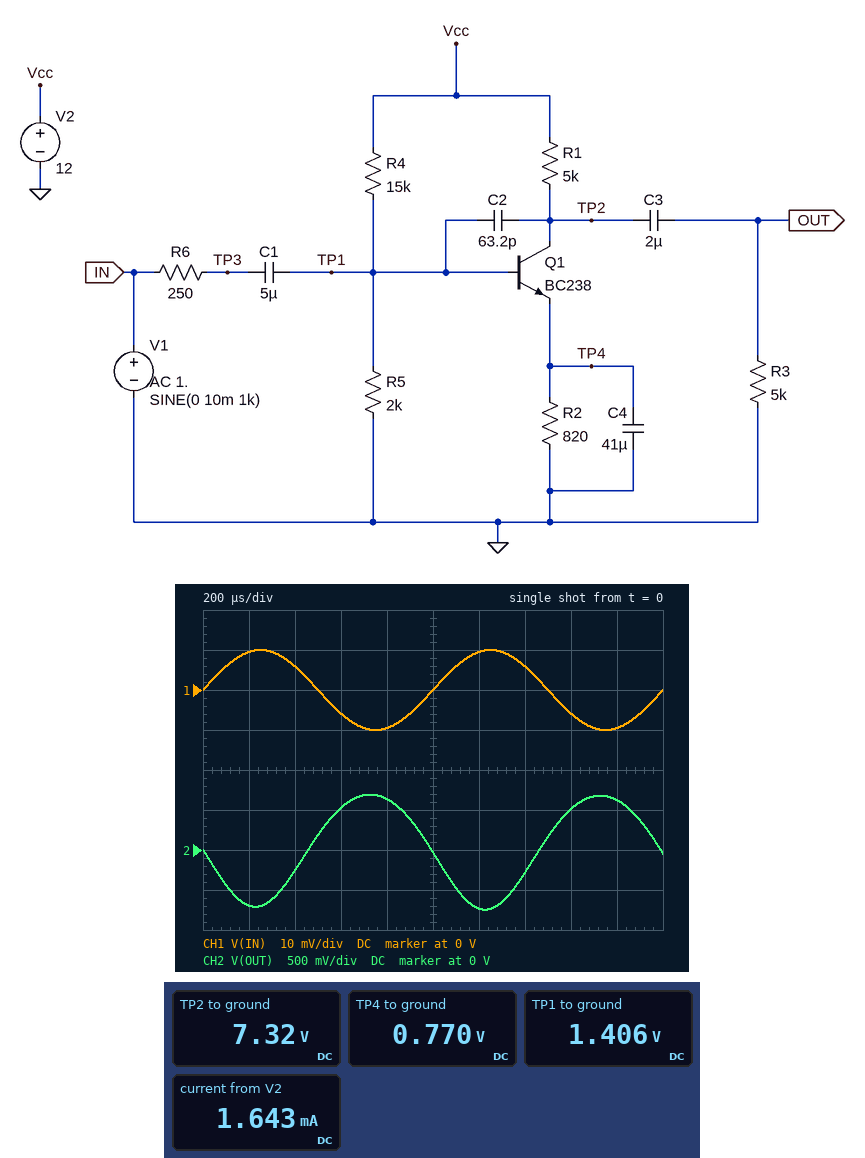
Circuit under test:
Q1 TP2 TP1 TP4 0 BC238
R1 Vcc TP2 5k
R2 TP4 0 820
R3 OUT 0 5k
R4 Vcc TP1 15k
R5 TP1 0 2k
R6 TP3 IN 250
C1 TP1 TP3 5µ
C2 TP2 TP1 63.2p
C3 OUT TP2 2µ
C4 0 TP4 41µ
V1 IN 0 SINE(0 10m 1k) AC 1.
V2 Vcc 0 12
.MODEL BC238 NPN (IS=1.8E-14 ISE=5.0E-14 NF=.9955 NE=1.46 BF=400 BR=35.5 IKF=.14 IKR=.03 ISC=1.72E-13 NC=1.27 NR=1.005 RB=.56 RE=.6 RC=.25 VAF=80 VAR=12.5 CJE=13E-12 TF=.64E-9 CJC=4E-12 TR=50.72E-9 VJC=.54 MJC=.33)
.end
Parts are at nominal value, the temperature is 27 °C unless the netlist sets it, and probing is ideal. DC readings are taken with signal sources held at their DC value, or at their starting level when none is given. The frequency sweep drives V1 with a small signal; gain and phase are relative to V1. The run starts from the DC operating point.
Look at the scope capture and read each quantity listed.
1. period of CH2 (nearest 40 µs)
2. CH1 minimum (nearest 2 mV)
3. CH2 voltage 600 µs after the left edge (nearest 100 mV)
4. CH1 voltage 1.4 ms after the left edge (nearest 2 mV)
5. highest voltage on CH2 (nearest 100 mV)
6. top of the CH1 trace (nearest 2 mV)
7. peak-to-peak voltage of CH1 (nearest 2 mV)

1.00 ms
-10 mV
500 mV
6 mV
700 mV
10 mV
20 mV
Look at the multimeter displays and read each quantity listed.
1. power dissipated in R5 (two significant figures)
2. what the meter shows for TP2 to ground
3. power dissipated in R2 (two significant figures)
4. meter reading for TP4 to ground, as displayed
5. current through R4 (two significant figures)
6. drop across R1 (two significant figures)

990 µW
7.32 V
720 µW
0.770 V
710 µA
4.7 V
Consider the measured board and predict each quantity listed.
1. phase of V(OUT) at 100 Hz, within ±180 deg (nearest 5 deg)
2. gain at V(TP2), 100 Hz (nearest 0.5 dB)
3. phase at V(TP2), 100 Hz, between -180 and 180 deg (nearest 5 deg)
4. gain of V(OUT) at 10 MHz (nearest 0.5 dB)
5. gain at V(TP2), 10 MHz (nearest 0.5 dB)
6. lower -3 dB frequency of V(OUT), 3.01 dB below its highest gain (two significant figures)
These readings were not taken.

-115 deg
32.5 dB
-125 deg
-1.5 dB
-1.5 dB
140 Hz
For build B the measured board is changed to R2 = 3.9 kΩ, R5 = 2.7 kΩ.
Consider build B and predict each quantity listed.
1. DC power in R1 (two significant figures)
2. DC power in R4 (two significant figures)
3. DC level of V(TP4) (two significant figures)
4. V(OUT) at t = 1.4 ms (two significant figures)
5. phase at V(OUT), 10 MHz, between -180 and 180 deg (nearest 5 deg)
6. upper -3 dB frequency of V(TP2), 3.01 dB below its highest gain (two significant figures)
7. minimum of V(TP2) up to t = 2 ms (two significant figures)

490 µW
6.9 mW
1.2 V
-130 mV
65 deg
260 kHz
10 V
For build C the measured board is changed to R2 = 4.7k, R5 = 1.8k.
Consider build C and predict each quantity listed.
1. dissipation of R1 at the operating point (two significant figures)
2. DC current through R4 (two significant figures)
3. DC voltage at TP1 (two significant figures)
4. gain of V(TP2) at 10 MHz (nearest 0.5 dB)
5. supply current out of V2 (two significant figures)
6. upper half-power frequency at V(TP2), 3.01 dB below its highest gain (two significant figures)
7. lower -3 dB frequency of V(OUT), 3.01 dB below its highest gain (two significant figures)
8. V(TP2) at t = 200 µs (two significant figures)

110 µW
710 µA
1.3 V
-4.0 dB
860 µA
420 kHz
33 Hz
11 V
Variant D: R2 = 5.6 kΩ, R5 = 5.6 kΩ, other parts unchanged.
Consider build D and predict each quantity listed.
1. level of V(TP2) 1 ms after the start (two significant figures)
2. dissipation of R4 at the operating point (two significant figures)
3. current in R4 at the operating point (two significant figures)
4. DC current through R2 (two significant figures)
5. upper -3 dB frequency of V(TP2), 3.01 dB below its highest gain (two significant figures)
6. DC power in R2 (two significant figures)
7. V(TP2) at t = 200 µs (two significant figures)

9.7 V
5.1 mW
580 µA
470 µA
190 kHz
1.2 mW
9.2 V
